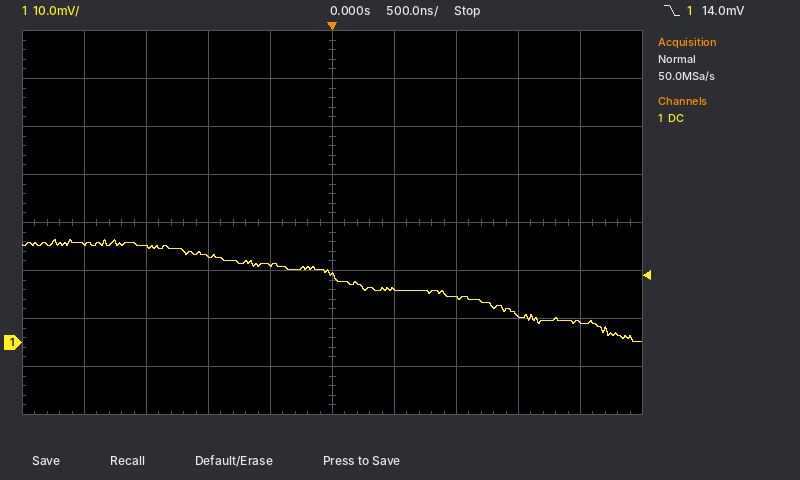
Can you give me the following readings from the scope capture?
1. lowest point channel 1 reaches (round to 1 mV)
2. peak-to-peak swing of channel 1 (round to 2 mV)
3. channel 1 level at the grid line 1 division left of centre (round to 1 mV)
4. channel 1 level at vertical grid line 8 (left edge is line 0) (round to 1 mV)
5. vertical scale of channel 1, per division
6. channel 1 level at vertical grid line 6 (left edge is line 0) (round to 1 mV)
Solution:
0 mV
22 mV
16 mV
6 mV
10 mV
11 mV
